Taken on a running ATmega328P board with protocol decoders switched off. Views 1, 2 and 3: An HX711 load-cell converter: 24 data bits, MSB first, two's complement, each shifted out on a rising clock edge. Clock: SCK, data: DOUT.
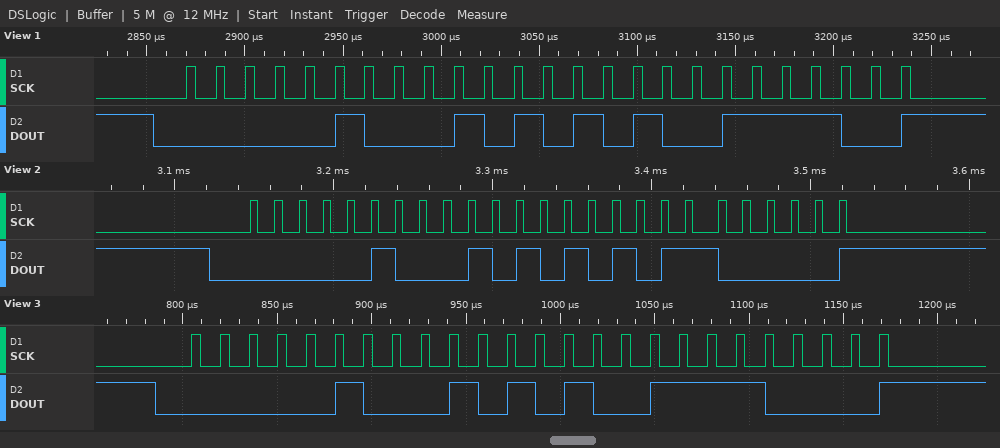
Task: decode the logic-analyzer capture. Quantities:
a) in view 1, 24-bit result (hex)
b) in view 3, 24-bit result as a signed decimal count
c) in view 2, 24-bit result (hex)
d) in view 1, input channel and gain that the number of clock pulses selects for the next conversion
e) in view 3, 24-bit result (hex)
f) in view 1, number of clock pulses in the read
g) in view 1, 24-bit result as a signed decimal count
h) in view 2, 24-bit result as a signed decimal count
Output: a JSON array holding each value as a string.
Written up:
["0x04553C", "283888", "0x045560", "channel A, gain 128", "0x0454F0", "25", "283964", "284000"]
